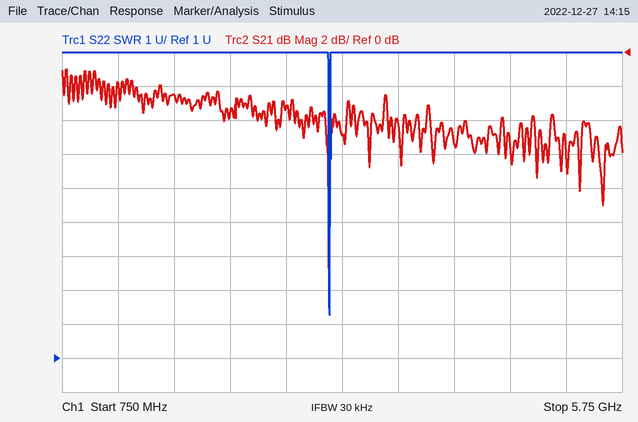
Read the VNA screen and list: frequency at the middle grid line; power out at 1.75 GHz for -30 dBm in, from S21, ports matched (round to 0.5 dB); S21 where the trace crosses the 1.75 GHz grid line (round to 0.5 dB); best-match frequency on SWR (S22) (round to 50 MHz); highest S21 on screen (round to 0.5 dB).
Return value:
3.25 GHz
-32.5 dBm
-2.5 dB
3.15 GHz
-1.0 dB
